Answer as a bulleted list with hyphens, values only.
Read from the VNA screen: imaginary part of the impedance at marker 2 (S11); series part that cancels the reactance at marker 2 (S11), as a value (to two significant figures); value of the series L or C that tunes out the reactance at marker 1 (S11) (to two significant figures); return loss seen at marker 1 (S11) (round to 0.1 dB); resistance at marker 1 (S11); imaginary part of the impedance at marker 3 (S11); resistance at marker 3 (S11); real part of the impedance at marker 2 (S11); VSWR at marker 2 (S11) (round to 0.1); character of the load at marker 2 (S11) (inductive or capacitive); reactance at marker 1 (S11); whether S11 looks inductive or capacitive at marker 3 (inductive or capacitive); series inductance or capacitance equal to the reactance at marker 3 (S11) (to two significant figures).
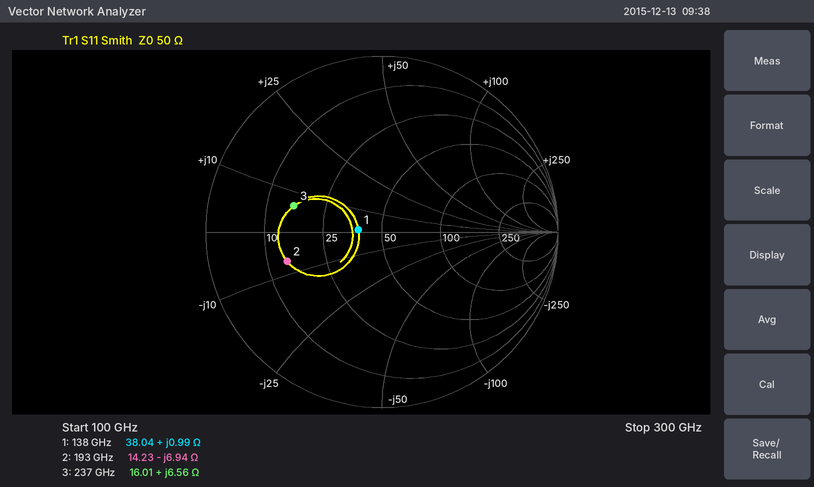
- -6.94 Ω
- 5.7 pH
- 1.2 pF
- 17.3 dB
- 38.04 Ω
- +6.56 Ω
- 16.01 Ω
- 14.23 Ω
- 3.6
- capacitive
- +0.99 Ω
- inductive
- 4.4 pH
